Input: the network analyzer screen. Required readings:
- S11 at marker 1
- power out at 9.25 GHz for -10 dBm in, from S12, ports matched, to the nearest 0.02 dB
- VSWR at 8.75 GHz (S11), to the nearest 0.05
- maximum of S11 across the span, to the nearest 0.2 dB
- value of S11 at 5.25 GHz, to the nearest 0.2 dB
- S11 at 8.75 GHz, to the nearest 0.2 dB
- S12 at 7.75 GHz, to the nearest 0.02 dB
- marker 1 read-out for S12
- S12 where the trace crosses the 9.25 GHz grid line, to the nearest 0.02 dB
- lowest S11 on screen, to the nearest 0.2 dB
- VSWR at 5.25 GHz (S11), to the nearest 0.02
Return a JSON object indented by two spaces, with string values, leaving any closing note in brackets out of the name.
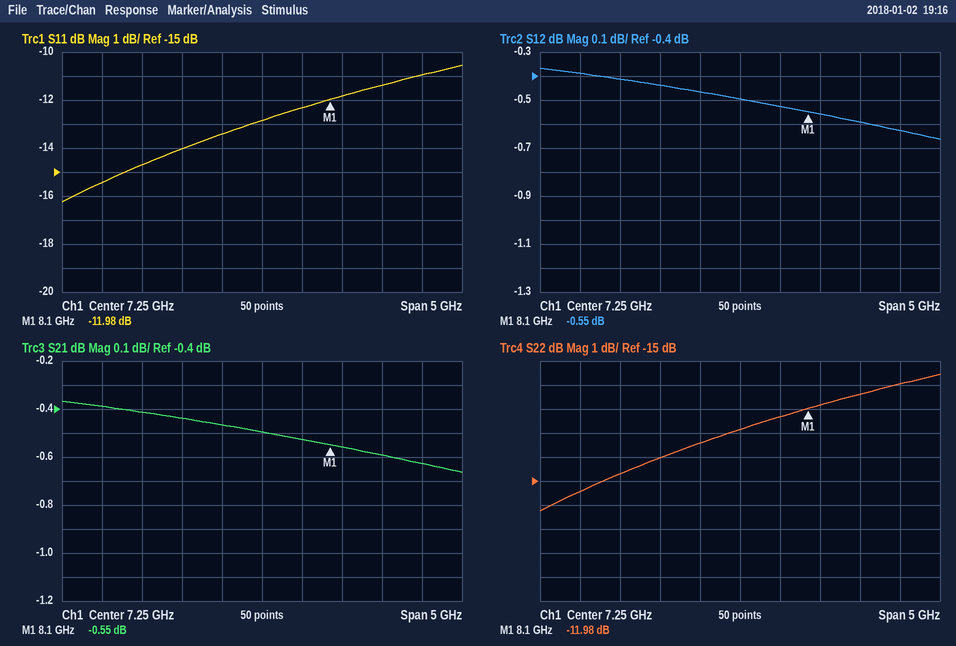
{
  "S11 at marker 1": "-11.98 dB",
  "power out at 9.25 GHz for -10 dBm in, from S12, ports matched, to the nearest 0.02 dB": "-10.62 dBm",
  "VSWR at 8.75 GHz (S11), to the nearest 0.05": "1.75",
  "maximum of S11 across the span, to the nearest 0.2 dB": "-10.6 dB",
  "value of S11 at 5.25 GHz, to the nearest 0.2 dB": "-15.4 dB",
  "S11 at 8.75 GHz, to the nearest 0.2 dB": "-11.4 dB",
  "S12 at 7.75 GHz, to the nearest 0.02 dB": "-0.52 dB",
  "marker 1 read-out for S12": "-0.55 dB",
  "S12 where the trace crosses the 9.25 GHz grid line, to the nearest 0.02 dB": "-0.62 dB",
  "lowest S11 on screen, to the nearest 0.2 dB": "-16.2 dB",
  "VSWR at 5.25 GHz (S11), to the nearest 0.02": "1.40"
}
